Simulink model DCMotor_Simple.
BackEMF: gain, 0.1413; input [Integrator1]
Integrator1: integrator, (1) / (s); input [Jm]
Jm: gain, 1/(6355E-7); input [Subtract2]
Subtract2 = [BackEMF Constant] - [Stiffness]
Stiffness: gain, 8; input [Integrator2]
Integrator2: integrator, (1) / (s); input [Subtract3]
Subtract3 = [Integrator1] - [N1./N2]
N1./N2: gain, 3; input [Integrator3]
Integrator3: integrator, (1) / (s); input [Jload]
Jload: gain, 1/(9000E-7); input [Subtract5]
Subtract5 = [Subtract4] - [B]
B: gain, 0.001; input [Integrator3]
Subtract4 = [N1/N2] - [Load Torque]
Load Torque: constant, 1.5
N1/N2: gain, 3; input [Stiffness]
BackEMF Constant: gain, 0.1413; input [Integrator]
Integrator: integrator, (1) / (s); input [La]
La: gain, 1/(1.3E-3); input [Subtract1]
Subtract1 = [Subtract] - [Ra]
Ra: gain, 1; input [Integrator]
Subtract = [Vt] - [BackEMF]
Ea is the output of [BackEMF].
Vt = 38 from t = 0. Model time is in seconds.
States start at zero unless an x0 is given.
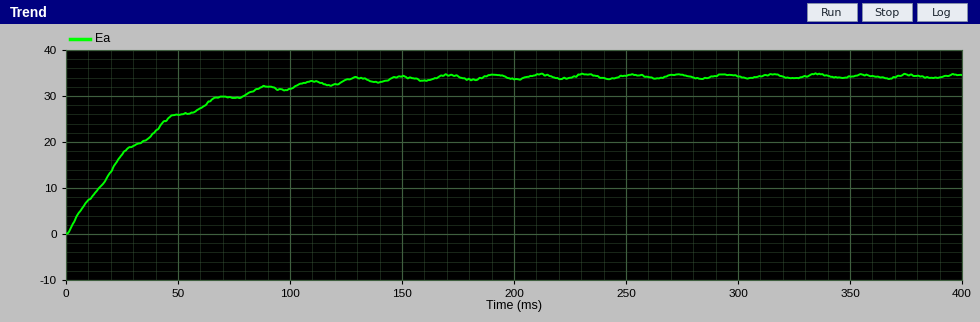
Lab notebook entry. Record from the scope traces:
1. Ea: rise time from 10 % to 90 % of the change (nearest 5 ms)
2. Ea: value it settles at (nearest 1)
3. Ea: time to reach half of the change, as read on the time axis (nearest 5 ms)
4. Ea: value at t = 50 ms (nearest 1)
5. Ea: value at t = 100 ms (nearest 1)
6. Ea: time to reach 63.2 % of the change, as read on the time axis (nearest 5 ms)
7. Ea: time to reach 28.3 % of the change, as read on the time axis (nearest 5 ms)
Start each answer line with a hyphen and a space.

- 80 ms
- 34
- 25 ms
- 26
- 32
- 40 ms
- 15 ms
